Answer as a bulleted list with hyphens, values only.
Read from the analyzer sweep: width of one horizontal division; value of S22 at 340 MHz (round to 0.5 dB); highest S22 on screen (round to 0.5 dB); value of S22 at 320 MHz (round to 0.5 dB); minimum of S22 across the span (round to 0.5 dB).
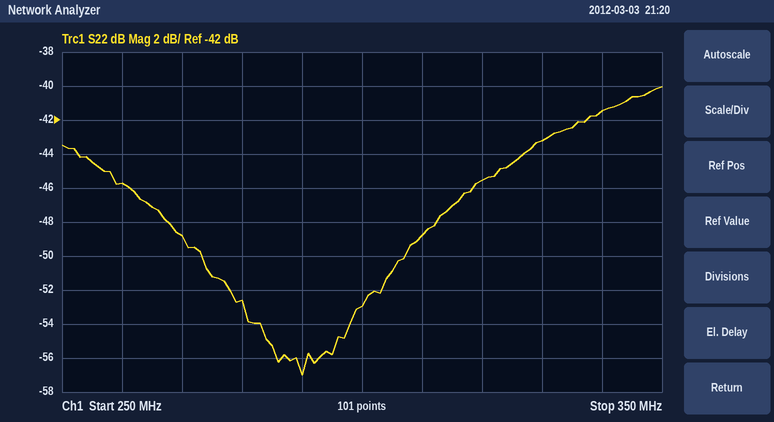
- 10 MHz
- -41.5 dB
- -40.0 dB
- -45.5 dB
- -57.0 dB
